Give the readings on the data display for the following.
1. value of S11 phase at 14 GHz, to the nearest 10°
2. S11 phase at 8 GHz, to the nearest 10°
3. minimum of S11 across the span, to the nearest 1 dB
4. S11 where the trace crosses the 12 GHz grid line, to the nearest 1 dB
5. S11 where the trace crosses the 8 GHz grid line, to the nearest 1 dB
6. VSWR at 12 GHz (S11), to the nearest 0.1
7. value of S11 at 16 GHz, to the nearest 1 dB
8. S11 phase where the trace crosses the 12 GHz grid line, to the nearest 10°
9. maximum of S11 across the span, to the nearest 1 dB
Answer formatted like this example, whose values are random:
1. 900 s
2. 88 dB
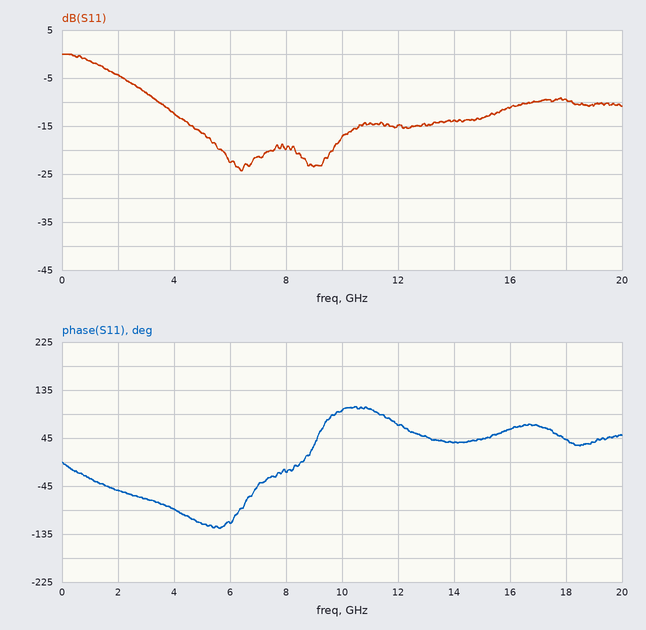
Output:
1. 40°
2. -20°
3. -24 dB
4. -15 dB
5. -20 dB
6. 1.4
7. -11 dB
8. 70°
9. 0 dB
